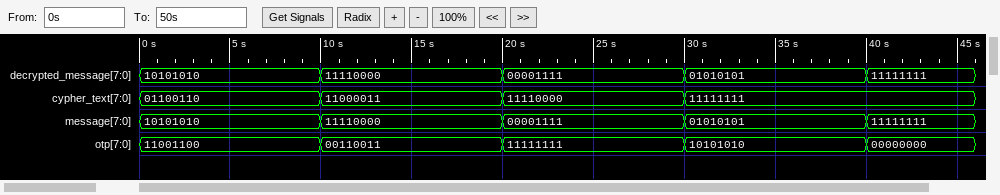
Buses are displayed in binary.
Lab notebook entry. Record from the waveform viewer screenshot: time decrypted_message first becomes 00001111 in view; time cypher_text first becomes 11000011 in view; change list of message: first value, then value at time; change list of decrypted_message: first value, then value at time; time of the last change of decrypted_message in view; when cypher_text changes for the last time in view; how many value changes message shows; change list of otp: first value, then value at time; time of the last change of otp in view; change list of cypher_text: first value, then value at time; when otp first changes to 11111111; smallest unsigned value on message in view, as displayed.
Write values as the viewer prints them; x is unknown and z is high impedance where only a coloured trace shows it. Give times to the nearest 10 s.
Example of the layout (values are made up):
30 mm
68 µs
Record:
20 s
10 s
10101010, 11110000 at 10 s, 00001111 at 20 s, 01010101 at 30 s, 11111111 at 40 s
10101010, 11110000 at 10 s, 00001111 at 20 s, 01010101 at 30 s, 11111111 at 40 s
40 s
30 s
4
11001100, 00110011 at 10 s, 11111111 at 20 s, 10101010 at 30 s, 00000000 at 40 s
40 s
01100110, 11000011 at 10 s, 11110000 at 20 s, 11111111 at 30 s
20 s
00001111
